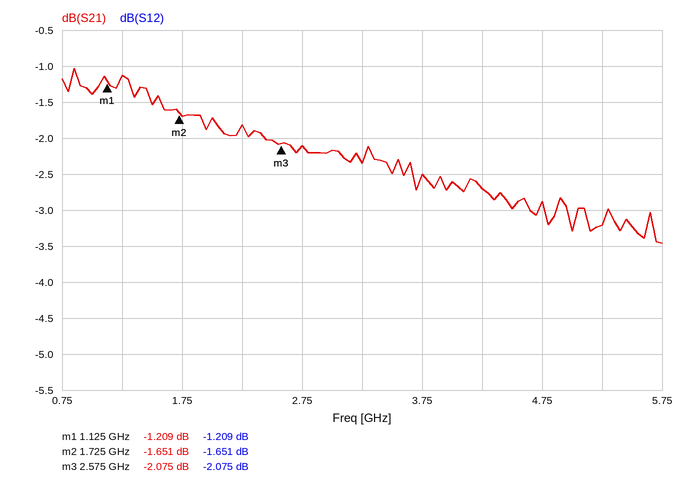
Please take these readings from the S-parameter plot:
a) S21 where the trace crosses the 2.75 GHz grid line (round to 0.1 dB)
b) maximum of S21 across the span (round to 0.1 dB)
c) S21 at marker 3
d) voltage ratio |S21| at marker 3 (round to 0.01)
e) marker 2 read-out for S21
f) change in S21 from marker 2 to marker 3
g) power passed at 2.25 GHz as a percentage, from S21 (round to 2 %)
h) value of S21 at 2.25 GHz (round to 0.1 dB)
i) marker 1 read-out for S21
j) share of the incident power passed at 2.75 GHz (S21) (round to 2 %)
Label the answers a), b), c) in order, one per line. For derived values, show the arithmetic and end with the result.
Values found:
a) -2.1 dB
b) -1.0 dB
c) -2.075 dB
d) 10^(-2.075/20) ≈ 0.79
e) -1.651 dB
f) -2.075 − (-1.651) = -0.424 dB
g) 10^(-1.8/10) ≈ 66 %
h) -1.8 dB
i) -1.209 dB
j) 10^(-2.1/10) ≈ 62 %
